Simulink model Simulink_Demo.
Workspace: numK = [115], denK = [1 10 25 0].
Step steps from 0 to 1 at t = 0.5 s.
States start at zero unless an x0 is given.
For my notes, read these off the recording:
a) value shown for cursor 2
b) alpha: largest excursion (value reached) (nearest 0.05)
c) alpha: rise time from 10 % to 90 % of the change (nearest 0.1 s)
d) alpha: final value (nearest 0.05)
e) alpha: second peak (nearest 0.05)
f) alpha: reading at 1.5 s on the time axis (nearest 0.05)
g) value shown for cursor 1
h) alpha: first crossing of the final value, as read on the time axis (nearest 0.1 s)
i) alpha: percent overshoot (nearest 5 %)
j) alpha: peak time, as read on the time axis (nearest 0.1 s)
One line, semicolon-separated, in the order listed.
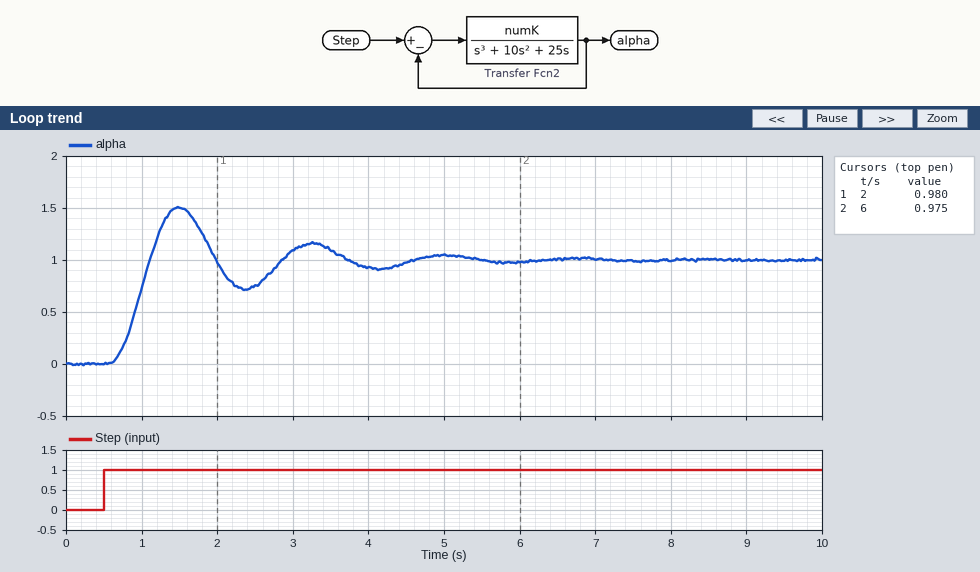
0.975; 1.50; 0.4 s; 1.00; 1.15; 1.50; 0.980; 1.1 s; 50 %; 1.5 s
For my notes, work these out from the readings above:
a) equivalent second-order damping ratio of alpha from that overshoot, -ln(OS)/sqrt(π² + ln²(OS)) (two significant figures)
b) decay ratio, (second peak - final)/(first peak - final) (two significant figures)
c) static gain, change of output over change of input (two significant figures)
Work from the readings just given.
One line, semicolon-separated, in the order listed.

0.22; 0.30; 1.0
